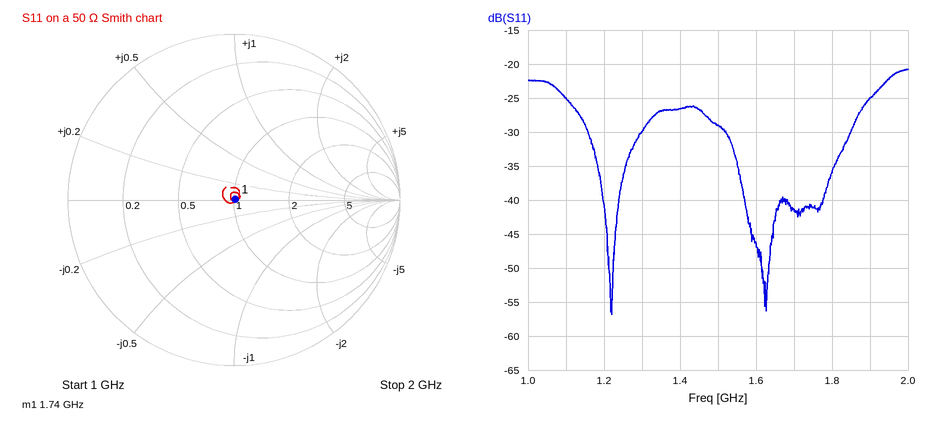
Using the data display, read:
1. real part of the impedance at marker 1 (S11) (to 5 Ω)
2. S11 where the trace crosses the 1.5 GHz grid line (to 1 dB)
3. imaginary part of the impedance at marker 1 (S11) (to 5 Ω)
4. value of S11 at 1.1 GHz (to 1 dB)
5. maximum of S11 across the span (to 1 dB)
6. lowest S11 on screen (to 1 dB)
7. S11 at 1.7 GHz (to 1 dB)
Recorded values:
50 Ω
-29 dB
0 Ω
-25 dB
-21 dB
-57 dB
-41 dB
